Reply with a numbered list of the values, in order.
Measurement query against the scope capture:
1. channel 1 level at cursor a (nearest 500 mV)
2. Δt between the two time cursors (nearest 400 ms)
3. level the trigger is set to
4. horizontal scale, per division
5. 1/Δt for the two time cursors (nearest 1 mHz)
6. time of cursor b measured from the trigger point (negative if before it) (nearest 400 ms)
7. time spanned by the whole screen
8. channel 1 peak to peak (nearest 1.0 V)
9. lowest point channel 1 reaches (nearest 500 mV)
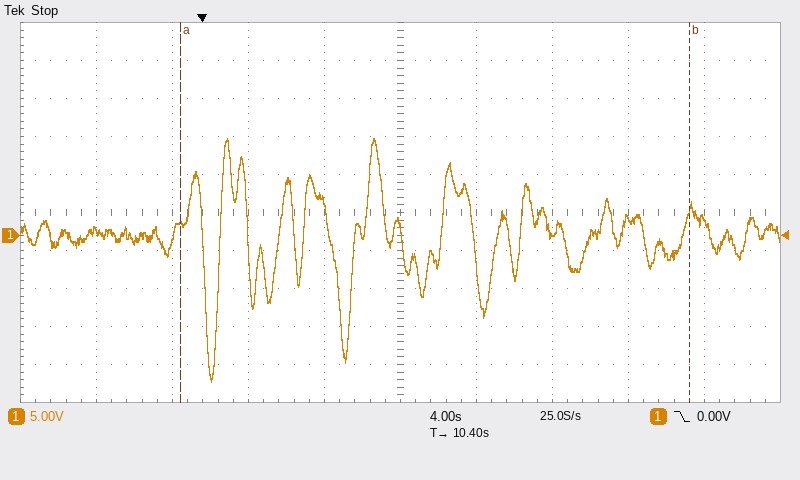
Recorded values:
1. 1.5 V
2. 26.8 s
3. 0.00 V
4. 4 s
5. 37 mHz
6. +25.6 s
7. 40 s
8. 32.0 V
9. -19.0 V
